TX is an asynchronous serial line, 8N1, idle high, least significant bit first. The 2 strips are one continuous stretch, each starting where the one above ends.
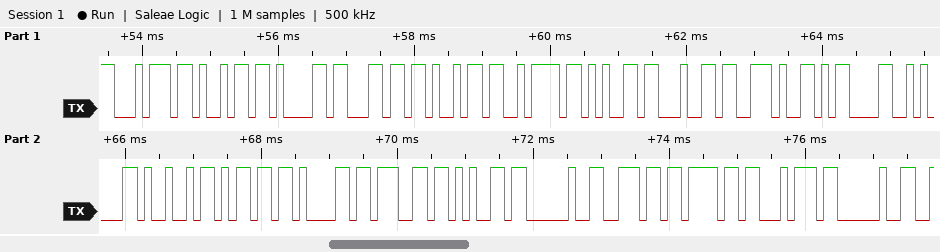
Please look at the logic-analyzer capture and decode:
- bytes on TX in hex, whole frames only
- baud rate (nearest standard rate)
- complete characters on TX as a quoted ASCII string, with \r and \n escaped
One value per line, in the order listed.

74 69 61 6C 69 7A 65 64 2E 0D 0A 49 6D 61 67 65 20 6E 6F 74 20
9600 baud
"tialized.\r\nImage not "
